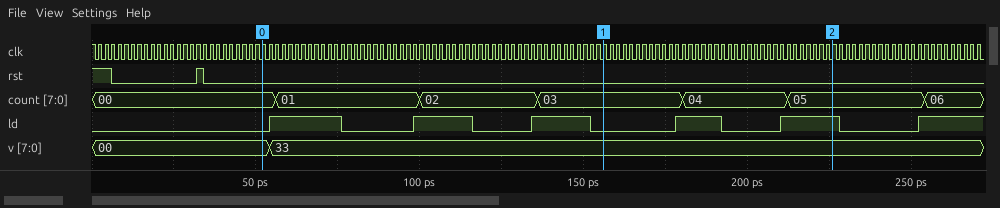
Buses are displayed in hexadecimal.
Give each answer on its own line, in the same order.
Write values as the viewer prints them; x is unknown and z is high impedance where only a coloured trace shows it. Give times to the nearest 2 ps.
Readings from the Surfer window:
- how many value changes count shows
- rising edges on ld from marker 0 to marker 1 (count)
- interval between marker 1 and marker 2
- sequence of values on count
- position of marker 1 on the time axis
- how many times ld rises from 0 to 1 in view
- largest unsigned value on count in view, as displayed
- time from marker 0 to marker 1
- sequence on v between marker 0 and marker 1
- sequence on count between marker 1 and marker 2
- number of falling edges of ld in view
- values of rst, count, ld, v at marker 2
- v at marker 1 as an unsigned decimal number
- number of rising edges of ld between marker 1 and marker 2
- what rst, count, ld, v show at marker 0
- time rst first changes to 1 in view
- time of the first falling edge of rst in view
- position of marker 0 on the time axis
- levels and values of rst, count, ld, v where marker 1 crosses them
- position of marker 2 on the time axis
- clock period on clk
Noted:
6
3
70 ps
00, 01, 02, 03, 04, 05, 06
156 ps
6
06
104 ps
00, 33
03, 04, 05
5
rst=0, count=05, ld=1, v=33
51
2
rst=0, count=00, ld=0, v=00
32 ps
6 ps
52 ps
rst=0, count=03, ld=0, v=33
226 ps
2 ps
